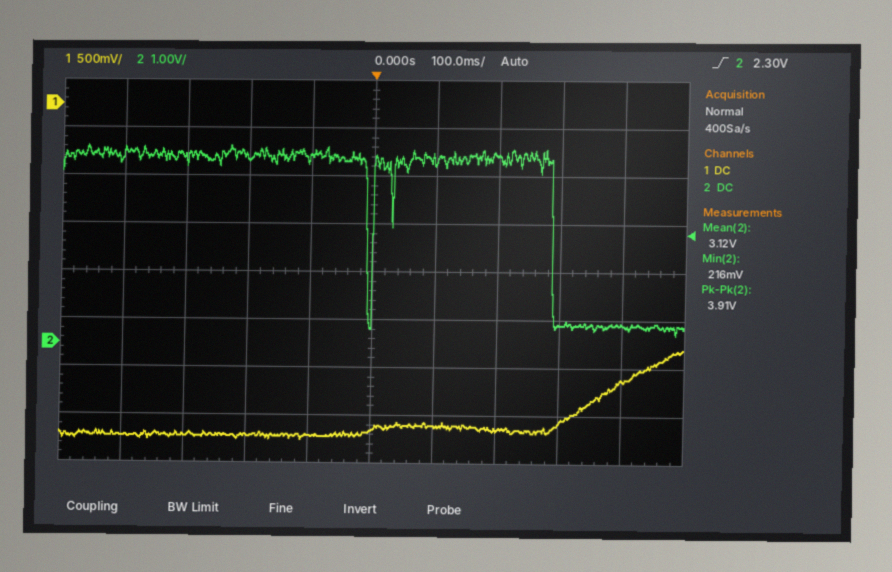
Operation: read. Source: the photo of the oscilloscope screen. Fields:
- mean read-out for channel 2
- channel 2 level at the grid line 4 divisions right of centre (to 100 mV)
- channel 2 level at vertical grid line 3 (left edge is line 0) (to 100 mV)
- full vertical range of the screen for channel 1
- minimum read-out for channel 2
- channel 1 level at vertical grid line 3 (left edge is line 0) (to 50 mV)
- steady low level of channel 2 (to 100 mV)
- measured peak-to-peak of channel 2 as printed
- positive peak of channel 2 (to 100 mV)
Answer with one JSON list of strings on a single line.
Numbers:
["3.12 V", "400 mV", "3.9 V", "4 V", "216 mV", "-3.45 V", "400 mV", "3.91 V", "4.1 V"]
